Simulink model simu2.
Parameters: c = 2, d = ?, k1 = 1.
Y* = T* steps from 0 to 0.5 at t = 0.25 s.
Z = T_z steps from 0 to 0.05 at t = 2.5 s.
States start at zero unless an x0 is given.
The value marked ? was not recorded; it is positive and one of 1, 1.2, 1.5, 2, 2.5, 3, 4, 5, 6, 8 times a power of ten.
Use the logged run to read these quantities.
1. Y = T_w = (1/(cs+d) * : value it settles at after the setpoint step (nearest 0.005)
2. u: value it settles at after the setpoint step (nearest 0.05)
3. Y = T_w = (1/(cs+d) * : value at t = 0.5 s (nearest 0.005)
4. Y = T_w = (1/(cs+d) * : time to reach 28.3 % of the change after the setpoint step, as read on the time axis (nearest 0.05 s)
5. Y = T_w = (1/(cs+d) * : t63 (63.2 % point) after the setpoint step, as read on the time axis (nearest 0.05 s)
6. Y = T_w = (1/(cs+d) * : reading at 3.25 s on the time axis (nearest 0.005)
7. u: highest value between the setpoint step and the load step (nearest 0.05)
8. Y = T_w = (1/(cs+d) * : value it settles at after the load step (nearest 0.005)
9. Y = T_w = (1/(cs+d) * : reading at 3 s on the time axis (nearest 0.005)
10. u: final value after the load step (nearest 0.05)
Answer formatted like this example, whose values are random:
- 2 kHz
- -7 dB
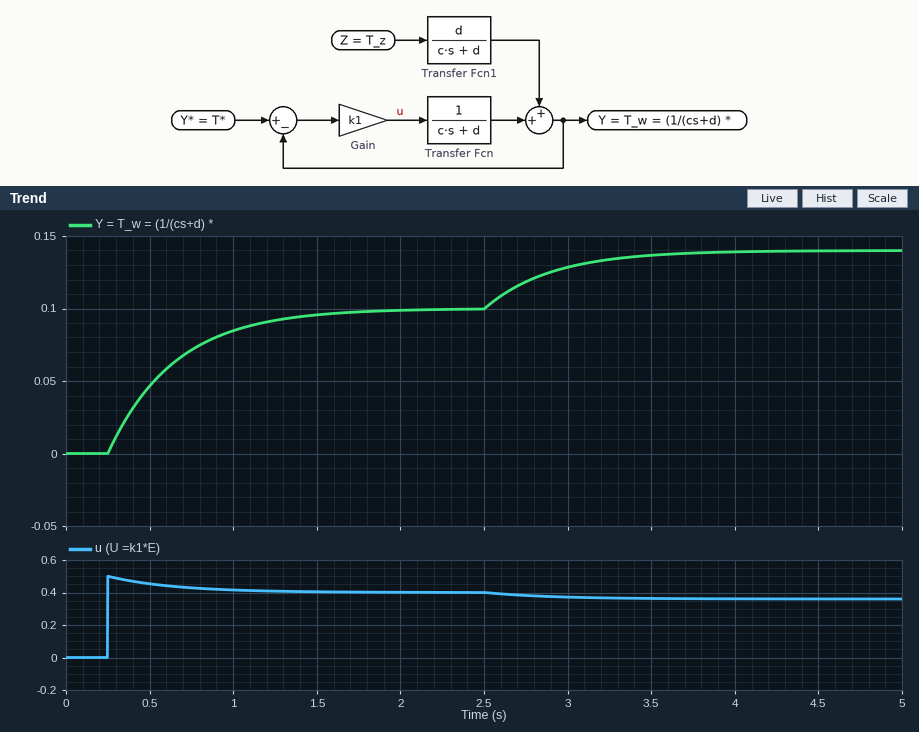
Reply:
- 0.100
- 0.40
- 0.045
- 0.40 s
- 0.65 s
- 0.135
- 0.50
- 0.140
- 0.130
- 0.35
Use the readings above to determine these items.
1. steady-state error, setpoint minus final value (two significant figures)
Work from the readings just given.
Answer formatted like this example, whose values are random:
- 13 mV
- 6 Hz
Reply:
- 0.40
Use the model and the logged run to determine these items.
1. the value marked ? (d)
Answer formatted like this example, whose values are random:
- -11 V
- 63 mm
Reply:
- 4
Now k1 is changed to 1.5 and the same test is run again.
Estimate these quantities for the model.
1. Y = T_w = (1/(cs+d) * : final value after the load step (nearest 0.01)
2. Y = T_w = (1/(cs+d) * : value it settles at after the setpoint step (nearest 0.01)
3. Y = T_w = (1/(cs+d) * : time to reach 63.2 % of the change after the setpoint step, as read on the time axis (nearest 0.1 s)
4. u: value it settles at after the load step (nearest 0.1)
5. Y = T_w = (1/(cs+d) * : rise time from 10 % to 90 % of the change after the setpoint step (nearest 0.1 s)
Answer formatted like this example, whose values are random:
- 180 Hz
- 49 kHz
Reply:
- 0.17
- 0.14
- 0.6 s
- 0.5
- 0.8 s
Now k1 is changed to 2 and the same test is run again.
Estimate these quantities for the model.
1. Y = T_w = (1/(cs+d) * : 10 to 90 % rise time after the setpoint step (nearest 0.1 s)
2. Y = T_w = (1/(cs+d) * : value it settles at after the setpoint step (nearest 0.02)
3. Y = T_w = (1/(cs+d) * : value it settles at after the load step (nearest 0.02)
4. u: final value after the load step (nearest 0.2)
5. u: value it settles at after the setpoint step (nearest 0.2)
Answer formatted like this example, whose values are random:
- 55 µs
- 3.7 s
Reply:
- 0.7 s
- 0.16
- 0.20
- 0.6
- 0.6
